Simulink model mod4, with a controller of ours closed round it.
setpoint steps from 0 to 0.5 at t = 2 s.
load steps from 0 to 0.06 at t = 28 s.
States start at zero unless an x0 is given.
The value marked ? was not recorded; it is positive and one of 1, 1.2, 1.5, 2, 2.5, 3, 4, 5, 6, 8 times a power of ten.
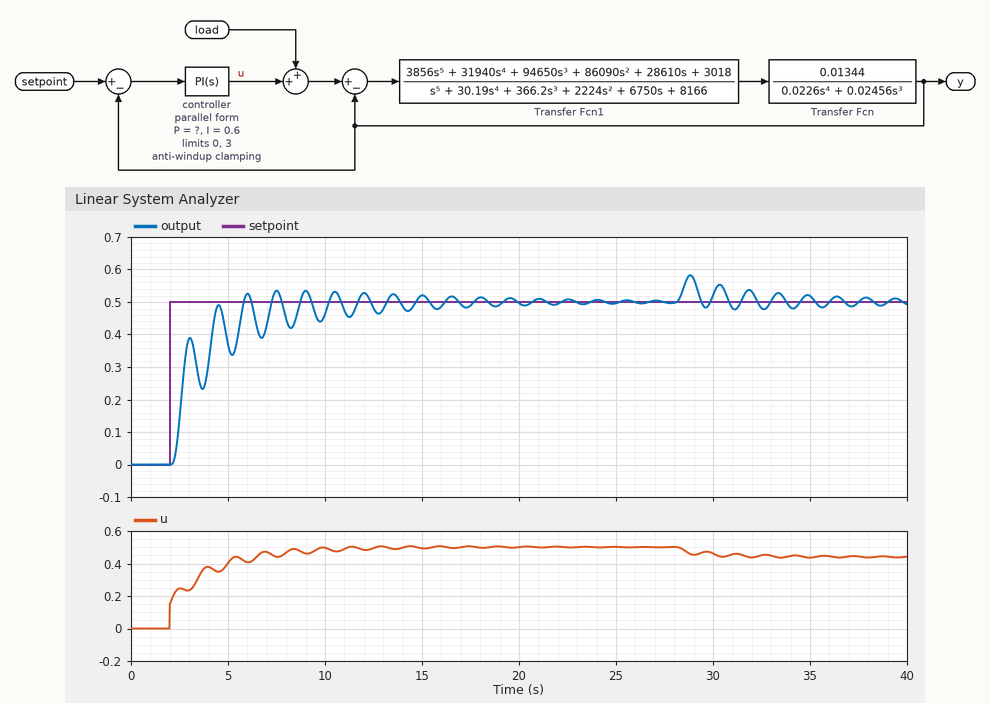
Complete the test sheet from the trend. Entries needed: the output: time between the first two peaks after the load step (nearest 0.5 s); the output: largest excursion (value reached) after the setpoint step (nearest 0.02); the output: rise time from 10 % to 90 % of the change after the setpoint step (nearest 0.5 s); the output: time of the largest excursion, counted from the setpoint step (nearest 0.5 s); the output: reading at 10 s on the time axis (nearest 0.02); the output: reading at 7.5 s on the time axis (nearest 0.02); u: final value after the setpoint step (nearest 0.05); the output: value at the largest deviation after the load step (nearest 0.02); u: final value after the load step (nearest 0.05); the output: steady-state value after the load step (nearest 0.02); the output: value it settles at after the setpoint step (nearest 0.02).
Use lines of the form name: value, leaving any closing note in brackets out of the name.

the output: time between the first two peaks after the load step: 1.5 s
the output: largest excursion (value reached) after the setpoint step: 0.54
the output: rise time from 10 % to 90 % of the change after the setpoint step: 2.0 s
the output: time of the largest excursion, counted from the setpoint step: 5.5 s
the output: reading at 10 s on the time axis: 0.46
the output: reading at 7.5 s on the time axis: 0.54
u: final value after the setpoint step: 0.50
the output: value at the largest deviation after the load step: 0.58
u: final value after the load step: 0.45
the output: steady-state value after the load step: 0.50
the output: value it settles at after the setpoint step: 0.50
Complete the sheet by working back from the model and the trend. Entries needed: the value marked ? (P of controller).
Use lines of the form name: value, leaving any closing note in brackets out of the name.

the value marked ?: 0.3
